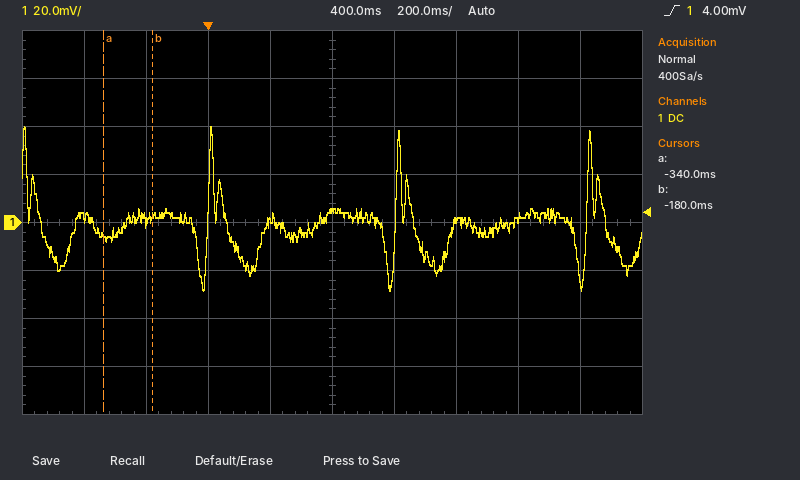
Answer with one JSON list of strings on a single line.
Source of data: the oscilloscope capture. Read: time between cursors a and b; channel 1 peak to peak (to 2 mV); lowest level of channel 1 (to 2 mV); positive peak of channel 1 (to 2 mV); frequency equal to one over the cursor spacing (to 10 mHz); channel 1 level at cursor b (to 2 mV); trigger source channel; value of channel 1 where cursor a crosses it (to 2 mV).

["160 ms", "68 mV", "-28 mV", "40 mV", "6.25 Hz", "2 mV", "channel 1", "-6 mV"]
